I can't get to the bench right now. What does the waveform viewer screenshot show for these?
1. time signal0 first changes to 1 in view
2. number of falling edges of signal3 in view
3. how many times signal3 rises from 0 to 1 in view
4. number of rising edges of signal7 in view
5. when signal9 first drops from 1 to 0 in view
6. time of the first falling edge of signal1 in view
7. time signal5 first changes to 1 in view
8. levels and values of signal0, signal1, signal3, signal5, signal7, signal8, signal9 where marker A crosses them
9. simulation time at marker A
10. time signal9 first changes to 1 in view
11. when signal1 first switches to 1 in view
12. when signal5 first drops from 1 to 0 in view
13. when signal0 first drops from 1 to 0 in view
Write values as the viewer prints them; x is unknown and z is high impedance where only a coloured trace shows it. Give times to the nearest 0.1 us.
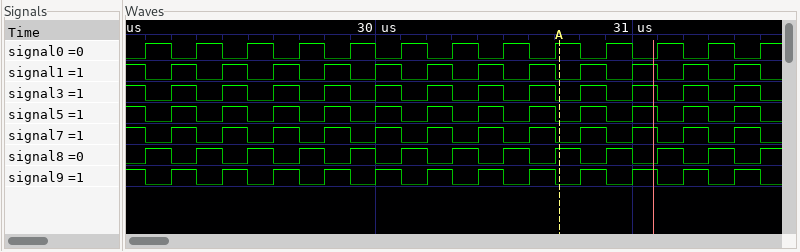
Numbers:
29.1 us
13
12
12
29.1 us
29.1 us
29.2 us
signal0=1, signal1=0, signal3=0, signal5=0, signal7=0, signal8=1, signal9=0
30.7 us
29.2 us
29.2 us
29.1 us
29.2 us
